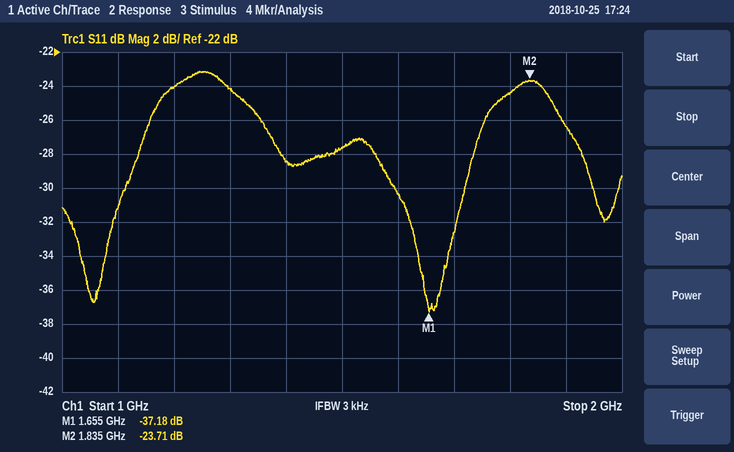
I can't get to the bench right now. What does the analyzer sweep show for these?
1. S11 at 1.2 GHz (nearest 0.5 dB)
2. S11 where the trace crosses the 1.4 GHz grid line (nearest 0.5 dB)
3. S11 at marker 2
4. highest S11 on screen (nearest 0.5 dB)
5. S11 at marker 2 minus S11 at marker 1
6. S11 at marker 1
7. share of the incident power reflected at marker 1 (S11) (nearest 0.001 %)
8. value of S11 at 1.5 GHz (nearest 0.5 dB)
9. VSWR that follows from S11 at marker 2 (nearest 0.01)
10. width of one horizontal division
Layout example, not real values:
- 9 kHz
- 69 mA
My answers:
- -24.0 dB
- -28.5 dB
- -23.71 dB
- -23.0 dB
- 13.47 dB
- -37.18 dB
- 0.019 %
- -27.5 dB
- 1.14
- 100 MHz
